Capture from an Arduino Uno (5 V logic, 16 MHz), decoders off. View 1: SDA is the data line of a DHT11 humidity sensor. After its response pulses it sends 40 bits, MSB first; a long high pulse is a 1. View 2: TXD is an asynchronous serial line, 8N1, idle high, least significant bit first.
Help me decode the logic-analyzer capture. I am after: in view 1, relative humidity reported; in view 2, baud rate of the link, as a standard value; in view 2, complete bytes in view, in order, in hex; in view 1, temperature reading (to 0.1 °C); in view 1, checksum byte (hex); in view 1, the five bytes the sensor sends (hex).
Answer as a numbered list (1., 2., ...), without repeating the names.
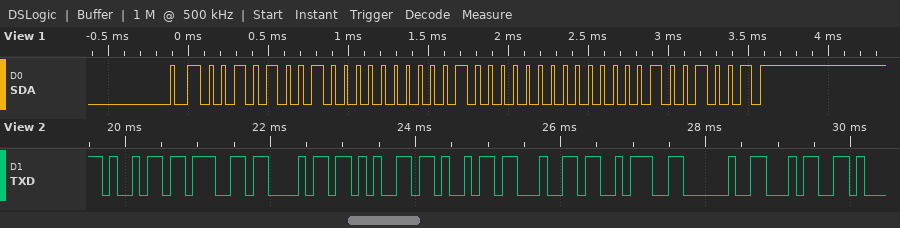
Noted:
1. 41 %
2. 9600 baud
3. 69 67 68 65 69 64 3A 20 34
4. 32.0 °C
5. 0x49
6. 29 00 20 00 49
